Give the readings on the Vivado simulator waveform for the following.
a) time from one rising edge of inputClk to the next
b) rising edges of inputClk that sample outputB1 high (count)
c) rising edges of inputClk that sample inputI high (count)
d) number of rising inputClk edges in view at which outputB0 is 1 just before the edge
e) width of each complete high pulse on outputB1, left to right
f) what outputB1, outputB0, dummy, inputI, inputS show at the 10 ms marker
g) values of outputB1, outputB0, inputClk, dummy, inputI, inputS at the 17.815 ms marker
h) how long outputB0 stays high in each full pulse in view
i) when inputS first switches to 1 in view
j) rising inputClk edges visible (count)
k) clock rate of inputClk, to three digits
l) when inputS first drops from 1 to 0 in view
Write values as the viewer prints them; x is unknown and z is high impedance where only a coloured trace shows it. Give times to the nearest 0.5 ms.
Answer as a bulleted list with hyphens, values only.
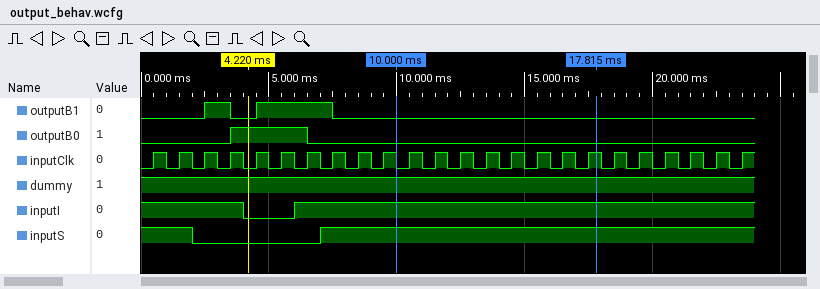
- 1 ms
- 4
- 22
- 3
- 1 ms, 3 ms
- outputB1=0, outputB0=0, dummy=1, inputI=1, inputS=1
- outputB1=0, outputB0=0, inputClk=1, dummy=1, inputI=1, inputS=1
- 3 ms
- 7 ms
- 24
- 1.00 kHz
- 2 ms
